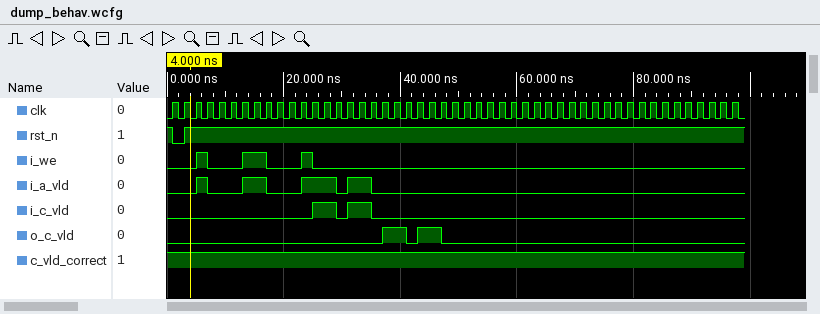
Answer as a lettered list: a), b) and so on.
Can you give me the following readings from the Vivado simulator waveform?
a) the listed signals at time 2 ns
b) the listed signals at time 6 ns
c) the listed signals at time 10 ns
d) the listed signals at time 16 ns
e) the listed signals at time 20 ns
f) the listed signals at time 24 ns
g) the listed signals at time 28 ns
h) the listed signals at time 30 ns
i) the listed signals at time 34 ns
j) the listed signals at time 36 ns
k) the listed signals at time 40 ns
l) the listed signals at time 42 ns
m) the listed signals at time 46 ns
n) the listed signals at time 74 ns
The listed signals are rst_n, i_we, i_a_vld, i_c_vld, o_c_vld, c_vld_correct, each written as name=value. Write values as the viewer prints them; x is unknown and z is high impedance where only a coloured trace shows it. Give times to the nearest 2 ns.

a) rst_n=0, i_we=0, i_a_vld=0, i_c_vld=0, o_c_vld=0, c_vld_correct=1
b) rst_n=1, i_we=1, i_a_vld=1, i_c_vld=0, o_c_vld=0, c_vld_correct=1
c) rst_n=1, i_we=0, i_a_vld=0, i_c_vld=0, o_c_vld=0, c_vld_correct=1
d) rst_n=1, i_we=1, i_a_vld=1, i_c_vld=0, o_c_vld=0, c_vld_correct=1
e) rst_n=1, i_we=0, i_a_vld=0, i_c_vld=0, o_c_vld=0, c_vld_correct=1
f) rst_n=1, i_we=1, i_a_vld=1, i_c_vld=0, o_c_vld=0, c_vld_correct=1
g) rst_n=1, i_we=0, i_a_vld=1, i_c_vld=1, o_c_vld=0, c_vld_correct=1
h) rst_n=1, i_we=0, i_a_vld=0, i_c_vld=0, o_c_vld=0, c_vld_correct=1
i) rst_n=1, i_we=0, i_a_vld=1, i_c_vld=1, o_c_vld=0, c_vld_correct=1
j) rst_n=1, i_we=0, i_a_vld=0, i_c_vld=0, o_c_vld=0, c_vld_correct=1
k) rst_n=1, i_we=0, i_a_vld=0, i_c_vld=0, o_c_vld=1, c_vld_correct=1
l) rst_n=1, i_we=0, i_a_vld=0, i_c_vld=0, o_c_vld=0, c_vld_correct=1
m) rst_n=1, i_we=0, i_a_vld=0, i_c_vld=0, o_c_vld=1, c_vld_correct=1
n) rst_n=1, i_we=0, i_a_vld=0, i_c_vld=0, o_c_vld=0, c_vld_correct=1
